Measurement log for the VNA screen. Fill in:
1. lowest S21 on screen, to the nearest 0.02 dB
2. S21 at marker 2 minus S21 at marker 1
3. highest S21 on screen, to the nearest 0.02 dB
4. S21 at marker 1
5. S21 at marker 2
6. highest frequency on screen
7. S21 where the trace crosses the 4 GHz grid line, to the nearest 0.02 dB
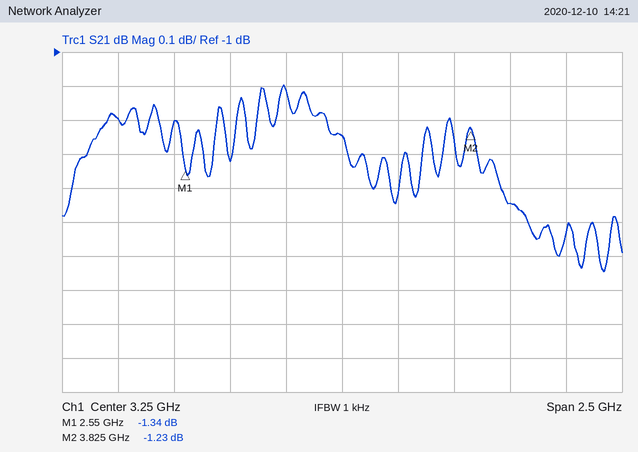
-1.64 dB
0.11 dB
-1.10 dB
-1.34 dB
-1.23 dB
4.5 GHz
-1.44 dB
